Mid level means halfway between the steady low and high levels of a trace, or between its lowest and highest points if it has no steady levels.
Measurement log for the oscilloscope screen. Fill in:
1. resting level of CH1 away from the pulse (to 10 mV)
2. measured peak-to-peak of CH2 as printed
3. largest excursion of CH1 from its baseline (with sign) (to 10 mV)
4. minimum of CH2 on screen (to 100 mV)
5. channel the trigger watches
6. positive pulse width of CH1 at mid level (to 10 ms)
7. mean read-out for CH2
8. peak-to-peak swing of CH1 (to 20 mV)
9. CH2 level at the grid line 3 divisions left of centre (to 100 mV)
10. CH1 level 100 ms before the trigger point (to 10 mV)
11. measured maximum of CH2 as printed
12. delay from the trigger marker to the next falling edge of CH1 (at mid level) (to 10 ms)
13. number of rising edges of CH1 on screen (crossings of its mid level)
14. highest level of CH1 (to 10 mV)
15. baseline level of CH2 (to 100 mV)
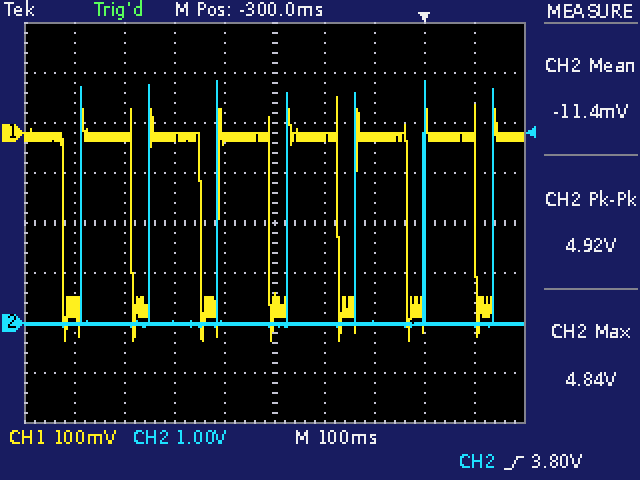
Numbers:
-10 mV
4.92 V
-410 mV
-100 mV
CH2
100 ms
-11.4 mV
480 mV
0.0 V
-10 mV
4.84 V
100 ms
7
70 mV
0.0 V
